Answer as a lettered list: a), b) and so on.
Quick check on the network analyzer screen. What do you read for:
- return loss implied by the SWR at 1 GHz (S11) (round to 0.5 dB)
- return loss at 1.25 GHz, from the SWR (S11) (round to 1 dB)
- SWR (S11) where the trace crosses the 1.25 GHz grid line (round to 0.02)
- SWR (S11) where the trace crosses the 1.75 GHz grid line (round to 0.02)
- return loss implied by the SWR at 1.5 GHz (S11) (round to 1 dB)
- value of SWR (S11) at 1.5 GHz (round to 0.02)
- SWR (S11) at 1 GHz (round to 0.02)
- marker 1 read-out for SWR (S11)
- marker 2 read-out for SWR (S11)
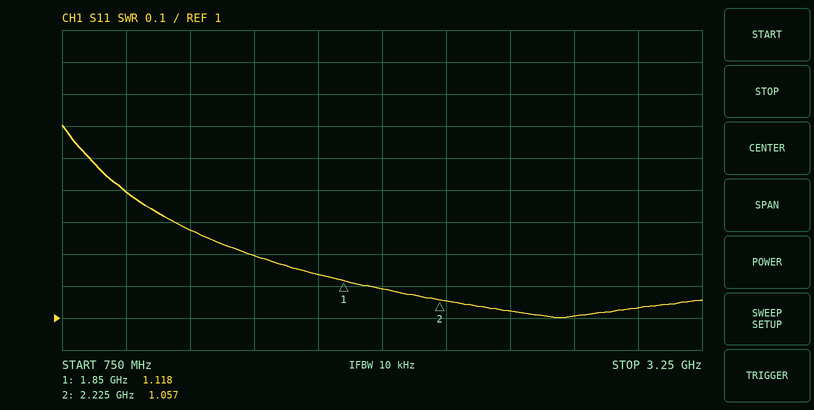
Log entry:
a) 15.5 dB
b) 18 dB
c) 1.28
d) 1.14
e) 21 dB
f) 1.20
g) 1.40
h) 1.118
i) 1.057
